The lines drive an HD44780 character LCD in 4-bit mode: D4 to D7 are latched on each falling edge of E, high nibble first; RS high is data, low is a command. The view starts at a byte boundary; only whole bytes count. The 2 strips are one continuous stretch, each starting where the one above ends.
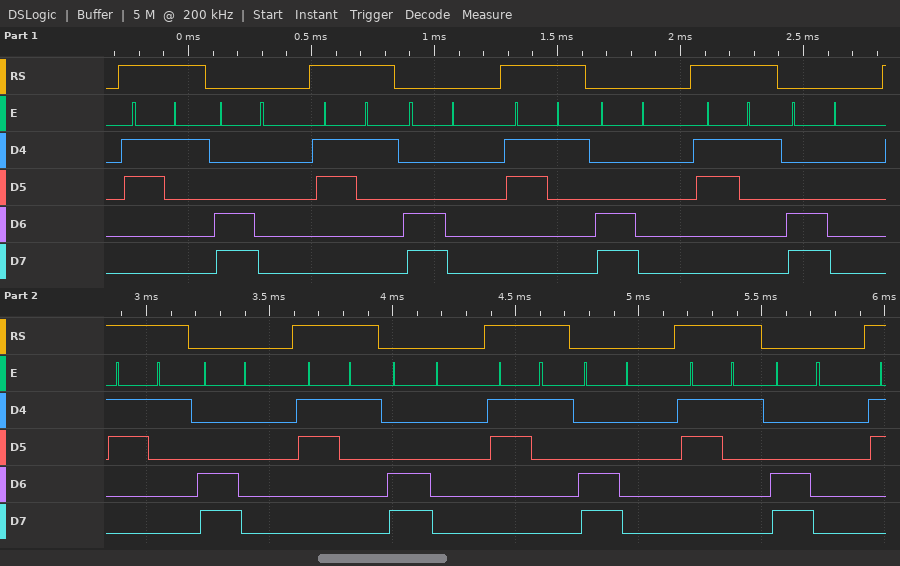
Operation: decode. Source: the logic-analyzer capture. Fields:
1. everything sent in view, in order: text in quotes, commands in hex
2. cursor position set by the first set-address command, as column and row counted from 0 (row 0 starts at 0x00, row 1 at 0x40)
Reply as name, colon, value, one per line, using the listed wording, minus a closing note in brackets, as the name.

everything sent in view, in order: text in quotes, commands in hex: "1" 0xC0 "1" 0xC0 "1" 0xC0 "1" 0xC0 "1" 0xC0 "1" 0xC0 "1" 0xC0 "1" 0xC0
cursor position set by the first set-address command, as column and row counted from 0: column 0, row 1
